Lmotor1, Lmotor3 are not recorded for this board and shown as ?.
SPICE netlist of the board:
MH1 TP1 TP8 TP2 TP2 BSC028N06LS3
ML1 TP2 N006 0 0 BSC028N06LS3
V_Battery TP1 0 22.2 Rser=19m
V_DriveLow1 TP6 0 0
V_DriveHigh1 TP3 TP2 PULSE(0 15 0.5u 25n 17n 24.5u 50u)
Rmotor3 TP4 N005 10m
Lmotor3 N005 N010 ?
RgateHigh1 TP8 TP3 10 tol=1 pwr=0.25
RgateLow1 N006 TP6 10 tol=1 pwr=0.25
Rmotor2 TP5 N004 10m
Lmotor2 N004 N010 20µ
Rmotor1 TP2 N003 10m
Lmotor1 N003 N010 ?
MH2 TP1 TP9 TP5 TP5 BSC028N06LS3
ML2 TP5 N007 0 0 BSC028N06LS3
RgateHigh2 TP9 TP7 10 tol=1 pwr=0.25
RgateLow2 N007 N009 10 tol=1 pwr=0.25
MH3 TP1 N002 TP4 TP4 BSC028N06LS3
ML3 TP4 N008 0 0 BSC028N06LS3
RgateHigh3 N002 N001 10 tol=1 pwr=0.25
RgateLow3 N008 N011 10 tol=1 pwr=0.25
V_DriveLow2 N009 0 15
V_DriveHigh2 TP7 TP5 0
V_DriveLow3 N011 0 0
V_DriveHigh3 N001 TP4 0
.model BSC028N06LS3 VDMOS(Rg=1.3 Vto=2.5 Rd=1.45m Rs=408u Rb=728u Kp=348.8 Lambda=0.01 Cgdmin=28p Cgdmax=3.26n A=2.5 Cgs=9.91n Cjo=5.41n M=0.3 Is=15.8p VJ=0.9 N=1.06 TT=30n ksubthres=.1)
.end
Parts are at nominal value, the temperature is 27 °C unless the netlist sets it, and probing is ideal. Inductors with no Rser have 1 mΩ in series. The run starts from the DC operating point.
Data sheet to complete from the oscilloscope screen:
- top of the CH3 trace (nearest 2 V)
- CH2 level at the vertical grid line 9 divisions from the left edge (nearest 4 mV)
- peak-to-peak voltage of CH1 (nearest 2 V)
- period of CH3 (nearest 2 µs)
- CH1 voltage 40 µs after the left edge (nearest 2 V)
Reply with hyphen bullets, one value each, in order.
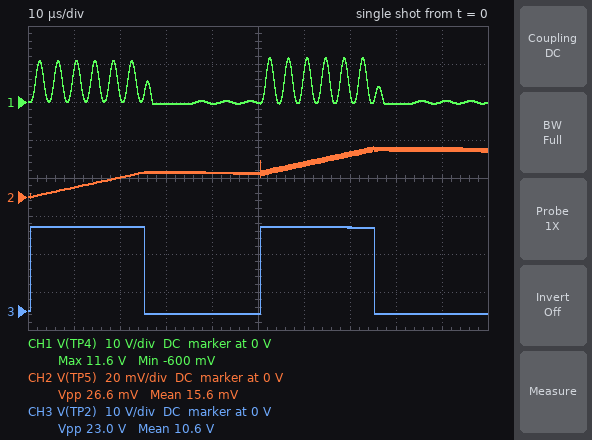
- 22 V
- 24 mV
- 12 V
- 50 µs
- 0 V
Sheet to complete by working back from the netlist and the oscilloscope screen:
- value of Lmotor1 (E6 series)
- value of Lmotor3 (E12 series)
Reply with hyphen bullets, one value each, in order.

- 68 µH
- 56 µH
